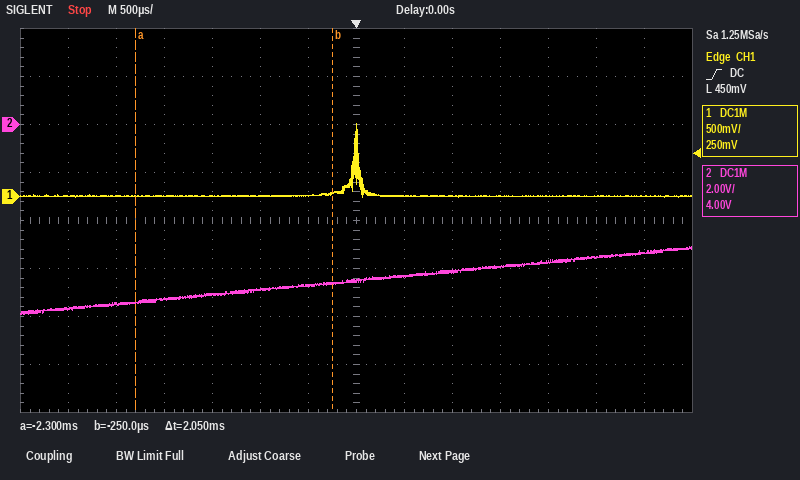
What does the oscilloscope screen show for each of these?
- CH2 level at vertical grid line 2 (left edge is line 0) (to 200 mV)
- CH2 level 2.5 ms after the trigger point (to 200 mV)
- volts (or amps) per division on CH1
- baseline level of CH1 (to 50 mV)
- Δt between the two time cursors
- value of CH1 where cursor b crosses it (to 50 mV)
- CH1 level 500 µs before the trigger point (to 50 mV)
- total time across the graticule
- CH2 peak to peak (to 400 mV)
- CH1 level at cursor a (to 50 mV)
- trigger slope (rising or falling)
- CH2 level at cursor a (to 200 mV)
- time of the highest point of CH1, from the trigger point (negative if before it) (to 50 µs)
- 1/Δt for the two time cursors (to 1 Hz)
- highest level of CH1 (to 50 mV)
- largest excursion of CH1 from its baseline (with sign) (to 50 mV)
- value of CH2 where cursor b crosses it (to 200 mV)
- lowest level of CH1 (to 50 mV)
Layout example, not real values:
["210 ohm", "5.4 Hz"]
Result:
["-7.4 V", "-5.6 V", "500 mV", "0 mV", "2.05 ms", "50 mV", "0 mV", "7 ms", "2.8 V", "0 mV", "rising", "-7.4 V", "0 µs", "488 Hz", "750 mV", "+750 mV", "-6.6 V", "0 mV"]
